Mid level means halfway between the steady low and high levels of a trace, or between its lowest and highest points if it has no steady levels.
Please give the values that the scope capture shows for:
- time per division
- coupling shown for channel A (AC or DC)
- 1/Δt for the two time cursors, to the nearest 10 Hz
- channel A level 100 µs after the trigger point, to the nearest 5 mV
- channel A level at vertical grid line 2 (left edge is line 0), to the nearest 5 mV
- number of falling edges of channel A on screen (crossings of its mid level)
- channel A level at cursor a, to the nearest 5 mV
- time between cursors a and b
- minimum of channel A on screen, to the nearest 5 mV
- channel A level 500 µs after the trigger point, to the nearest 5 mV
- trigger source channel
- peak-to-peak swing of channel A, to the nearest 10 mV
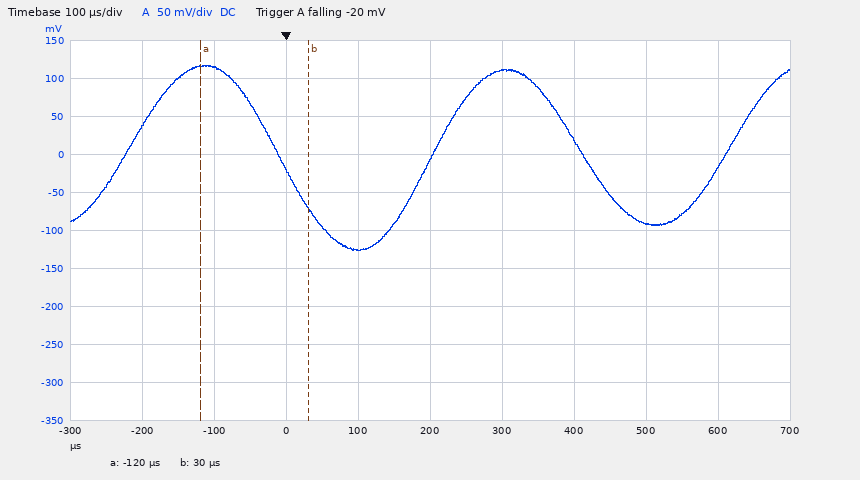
100 µs
DC
6.67 kHz
-125 mV
115 mV
2
115 mV
150 µs
-125 mV
-90 mV
channel A
240 mV
